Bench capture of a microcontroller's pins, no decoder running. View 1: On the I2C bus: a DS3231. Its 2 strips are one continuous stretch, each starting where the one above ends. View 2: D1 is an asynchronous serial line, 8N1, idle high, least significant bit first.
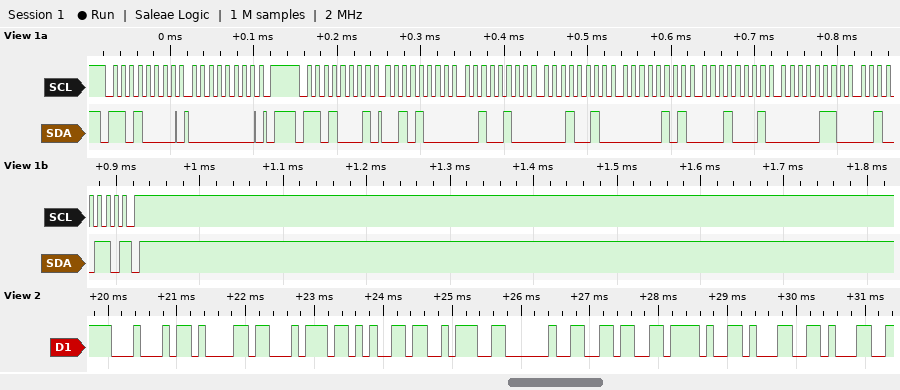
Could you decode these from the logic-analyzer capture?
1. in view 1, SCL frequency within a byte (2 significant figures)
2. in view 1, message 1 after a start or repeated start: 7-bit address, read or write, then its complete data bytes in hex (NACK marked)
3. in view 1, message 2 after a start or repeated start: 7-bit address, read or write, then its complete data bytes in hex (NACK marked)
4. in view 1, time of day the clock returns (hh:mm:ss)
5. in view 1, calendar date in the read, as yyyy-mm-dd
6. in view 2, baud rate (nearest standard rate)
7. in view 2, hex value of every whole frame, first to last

100 kHz
0x68 write: 00
0x68 read: 28 24 12 05 11 06 26 NACK
12:24:28
2026-06-11
9600 baud
44 61 74 65 3A 20 36 2F 31 31
